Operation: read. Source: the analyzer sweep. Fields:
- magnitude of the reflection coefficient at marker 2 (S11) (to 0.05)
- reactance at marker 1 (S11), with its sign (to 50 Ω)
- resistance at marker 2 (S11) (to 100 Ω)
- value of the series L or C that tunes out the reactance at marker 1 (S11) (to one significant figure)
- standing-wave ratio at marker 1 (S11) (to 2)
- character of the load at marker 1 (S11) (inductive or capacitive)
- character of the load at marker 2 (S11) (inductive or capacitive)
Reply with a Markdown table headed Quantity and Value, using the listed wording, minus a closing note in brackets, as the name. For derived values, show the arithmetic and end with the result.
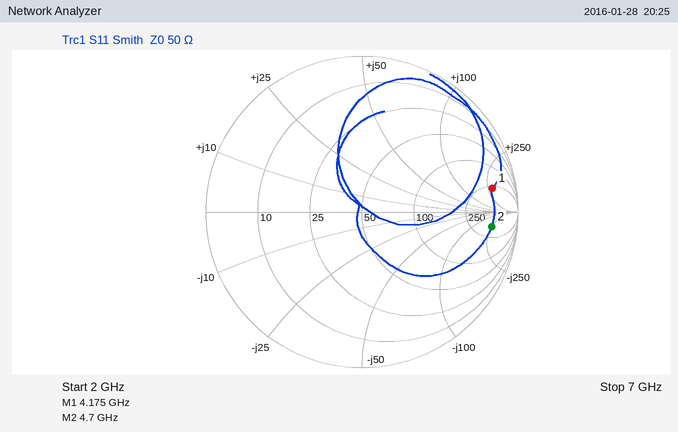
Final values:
| Quantity | Value |
|---|---|
| magnitude of the reflection coefficient at marker 2 (S11) | 0.85 |
| reactance at marker 1 (S11), with its sign | +300 Ω |
| resistance at marker 2 (S11) | 400 Ω |
| value of the series L or C that tunes out the reactance at marker 1 (S11) | C = 1/(2π × 4.175 GHz × 300 Ω) ≈ 127 fF, so 100 fF to one significant figure |
| standing-wave ratio at marker 1 (S11) | 12 |
| character of the load at marker 1 (S11) | inductive |
| character of the load at marker 2 (S11) | capacitive |
